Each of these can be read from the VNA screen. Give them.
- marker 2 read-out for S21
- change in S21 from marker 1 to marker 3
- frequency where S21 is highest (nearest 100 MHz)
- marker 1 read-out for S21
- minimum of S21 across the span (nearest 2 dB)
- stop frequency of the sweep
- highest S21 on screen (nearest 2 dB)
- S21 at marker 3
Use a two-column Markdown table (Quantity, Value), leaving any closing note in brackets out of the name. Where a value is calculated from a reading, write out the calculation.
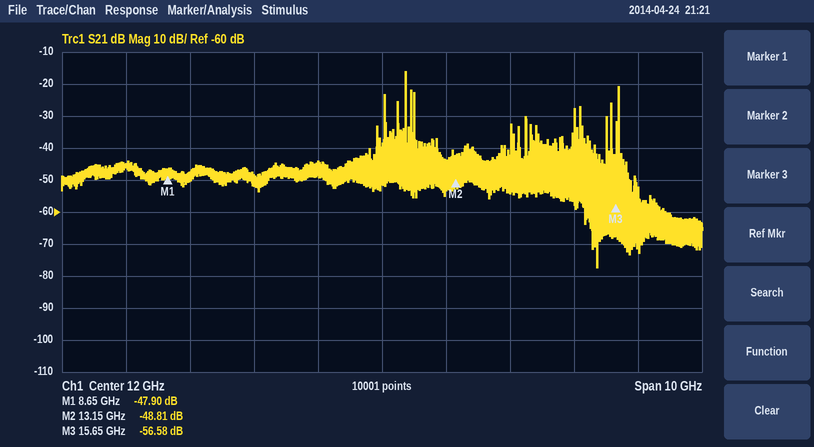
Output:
| Quantity | Value |
|---|---|
| marker 2 read-out for S21 | -48.81 dB |
| change in S21 from marker 1 to marker 3 | -56.58 − (-47.9) = -8.68 dB |
| frequency where S21 is highest | 12.4 GHz |
| marker 1 read-out for S21 | -47.90 dB |
| minimum of S21 across the span | -78 dB |
| stop frequency of the sweep | 17 GHz |
| highest S21 on screen | -16 dB |
| S21 at marker 3 | -56.58 dB |
